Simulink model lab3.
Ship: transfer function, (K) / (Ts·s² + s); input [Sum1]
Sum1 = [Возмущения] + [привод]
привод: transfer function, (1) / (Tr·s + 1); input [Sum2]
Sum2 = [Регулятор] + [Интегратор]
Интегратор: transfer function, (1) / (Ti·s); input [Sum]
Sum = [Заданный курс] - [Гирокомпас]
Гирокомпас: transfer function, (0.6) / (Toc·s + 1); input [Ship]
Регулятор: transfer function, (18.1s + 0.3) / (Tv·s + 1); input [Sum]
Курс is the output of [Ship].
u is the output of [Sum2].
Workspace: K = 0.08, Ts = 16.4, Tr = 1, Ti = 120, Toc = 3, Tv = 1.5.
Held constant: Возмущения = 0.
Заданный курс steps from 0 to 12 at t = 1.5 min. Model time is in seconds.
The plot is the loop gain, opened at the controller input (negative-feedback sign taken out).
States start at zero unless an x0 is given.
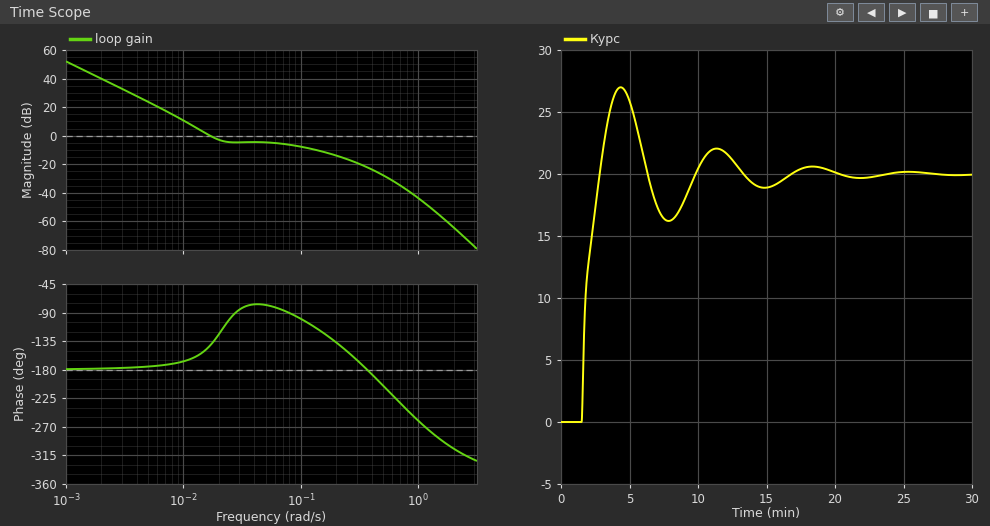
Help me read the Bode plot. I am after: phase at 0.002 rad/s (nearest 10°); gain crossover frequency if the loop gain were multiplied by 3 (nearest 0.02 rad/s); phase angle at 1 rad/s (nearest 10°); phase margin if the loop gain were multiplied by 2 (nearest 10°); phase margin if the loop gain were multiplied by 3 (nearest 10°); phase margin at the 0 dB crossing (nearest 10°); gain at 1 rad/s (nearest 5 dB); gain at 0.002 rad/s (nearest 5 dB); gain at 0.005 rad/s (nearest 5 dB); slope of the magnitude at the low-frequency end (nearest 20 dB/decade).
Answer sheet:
-180°
0.12 rad/s
-260°
90°
70°
40°
-45 dB
40 dB
25 dB
-40 dB/decade
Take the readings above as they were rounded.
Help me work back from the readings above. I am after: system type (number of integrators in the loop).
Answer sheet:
2
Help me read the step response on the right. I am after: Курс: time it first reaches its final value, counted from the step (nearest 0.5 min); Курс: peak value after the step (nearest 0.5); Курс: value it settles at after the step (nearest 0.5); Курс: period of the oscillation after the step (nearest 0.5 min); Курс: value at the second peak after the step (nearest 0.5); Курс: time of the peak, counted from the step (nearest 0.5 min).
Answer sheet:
1.5 min
27.0
20.0
7.0 min
22.0
3.0 min
